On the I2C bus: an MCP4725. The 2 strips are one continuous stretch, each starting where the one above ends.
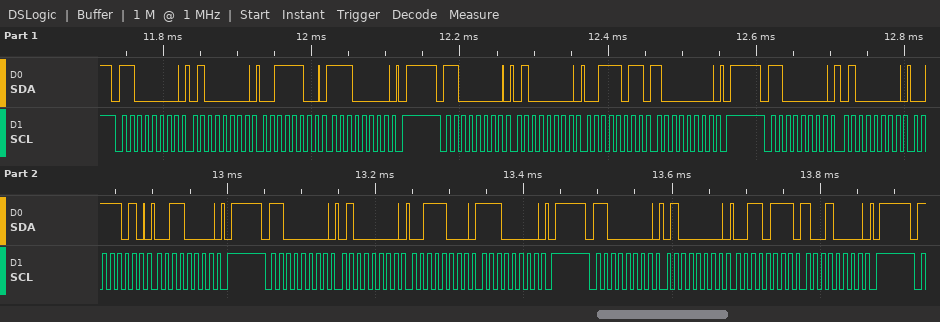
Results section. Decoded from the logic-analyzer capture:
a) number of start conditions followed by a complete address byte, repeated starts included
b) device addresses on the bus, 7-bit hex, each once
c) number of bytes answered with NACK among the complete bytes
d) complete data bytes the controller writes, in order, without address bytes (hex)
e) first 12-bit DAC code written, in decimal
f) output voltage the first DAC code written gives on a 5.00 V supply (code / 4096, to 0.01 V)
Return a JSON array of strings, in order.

["5", "0x60", "0", "40 3C E0 40 3B 80 40 3A 30 40 38 E0 40 37 90", "974", "1.19 V"]
